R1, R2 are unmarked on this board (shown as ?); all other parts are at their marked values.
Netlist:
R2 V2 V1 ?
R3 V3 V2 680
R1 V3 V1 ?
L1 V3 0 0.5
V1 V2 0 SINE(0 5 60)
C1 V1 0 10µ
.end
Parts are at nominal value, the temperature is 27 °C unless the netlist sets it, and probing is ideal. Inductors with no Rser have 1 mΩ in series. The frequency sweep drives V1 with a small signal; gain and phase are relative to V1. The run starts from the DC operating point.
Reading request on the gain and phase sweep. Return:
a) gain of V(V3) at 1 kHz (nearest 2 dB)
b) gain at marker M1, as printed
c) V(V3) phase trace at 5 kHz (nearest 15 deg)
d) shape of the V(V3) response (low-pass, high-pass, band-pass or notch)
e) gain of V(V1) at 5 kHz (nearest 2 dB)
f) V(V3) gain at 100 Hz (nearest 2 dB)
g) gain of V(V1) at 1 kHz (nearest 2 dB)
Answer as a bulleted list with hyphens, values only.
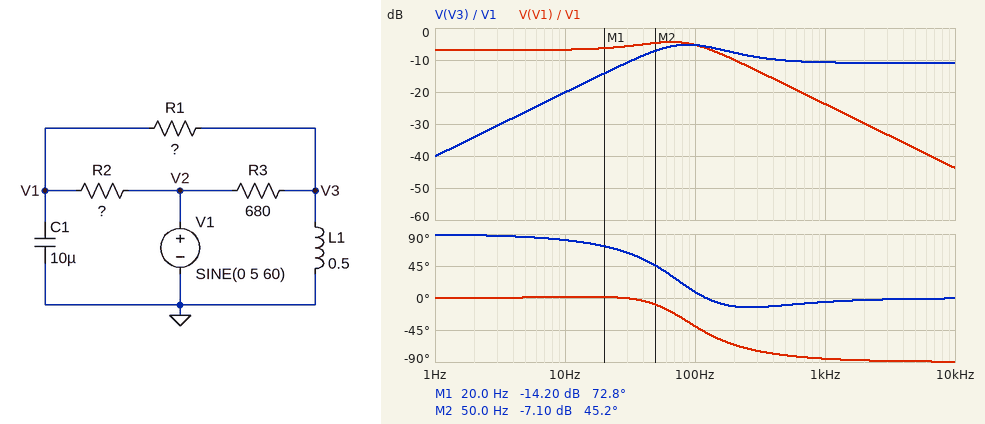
- -10 dB
- -14.20 dB
- 0 deg
- high-pass
- -38 dB
- -6 dB
- -24 dB
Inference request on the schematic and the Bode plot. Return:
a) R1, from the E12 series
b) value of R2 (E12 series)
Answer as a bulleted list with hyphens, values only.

- 270 Ω
- 330 Ω
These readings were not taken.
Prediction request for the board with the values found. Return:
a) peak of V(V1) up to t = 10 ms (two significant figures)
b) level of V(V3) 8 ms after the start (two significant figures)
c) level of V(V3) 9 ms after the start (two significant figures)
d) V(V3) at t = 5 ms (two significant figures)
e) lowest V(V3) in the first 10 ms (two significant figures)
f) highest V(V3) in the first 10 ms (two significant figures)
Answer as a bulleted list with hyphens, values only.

- 2.7 V
- -1.2 V
- -1.9 V
- 1.1 V
- -2.3 V
- 1.6 V
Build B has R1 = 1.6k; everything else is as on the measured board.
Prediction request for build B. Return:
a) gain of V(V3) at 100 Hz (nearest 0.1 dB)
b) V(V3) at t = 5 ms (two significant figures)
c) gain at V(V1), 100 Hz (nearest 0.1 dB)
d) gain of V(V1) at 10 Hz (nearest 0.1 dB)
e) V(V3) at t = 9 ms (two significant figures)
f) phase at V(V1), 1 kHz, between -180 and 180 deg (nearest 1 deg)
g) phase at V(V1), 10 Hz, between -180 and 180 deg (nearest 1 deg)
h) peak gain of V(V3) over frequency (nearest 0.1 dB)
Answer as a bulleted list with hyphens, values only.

- -7.3 dB
- 250 mV
- -7.1 dB
- -1.7 dB
- -1.5 V
- -86 deg
- -9 deg
- -3.1 dB
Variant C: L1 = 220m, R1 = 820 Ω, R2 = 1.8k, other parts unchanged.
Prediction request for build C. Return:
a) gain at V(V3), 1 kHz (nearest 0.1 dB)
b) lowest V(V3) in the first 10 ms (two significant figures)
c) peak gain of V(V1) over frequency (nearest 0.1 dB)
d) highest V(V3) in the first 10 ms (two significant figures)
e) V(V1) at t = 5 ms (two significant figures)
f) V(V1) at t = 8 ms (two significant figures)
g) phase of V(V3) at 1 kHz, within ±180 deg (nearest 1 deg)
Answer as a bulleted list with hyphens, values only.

- -5.5 dB
- -650 mV
- -10.1 dB
- 550 mV
- 840 mV
- 750 mV
- 14 deg
